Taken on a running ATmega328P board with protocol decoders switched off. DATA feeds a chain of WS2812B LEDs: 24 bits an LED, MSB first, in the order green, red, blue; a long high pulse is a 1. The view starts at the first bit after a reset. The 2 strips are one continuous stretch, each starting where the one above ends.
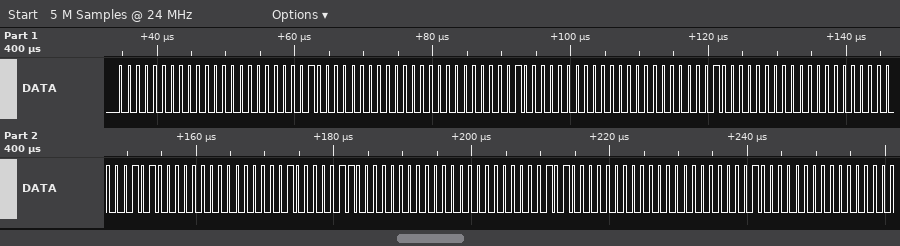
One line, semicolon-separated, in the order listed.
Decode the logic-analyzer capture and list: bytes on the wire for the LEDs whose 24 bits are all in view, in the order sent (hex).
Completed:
00 00 02 00 00 02 00 00 04 00 00 05 00 01 06 00 00 05 00 00 04
